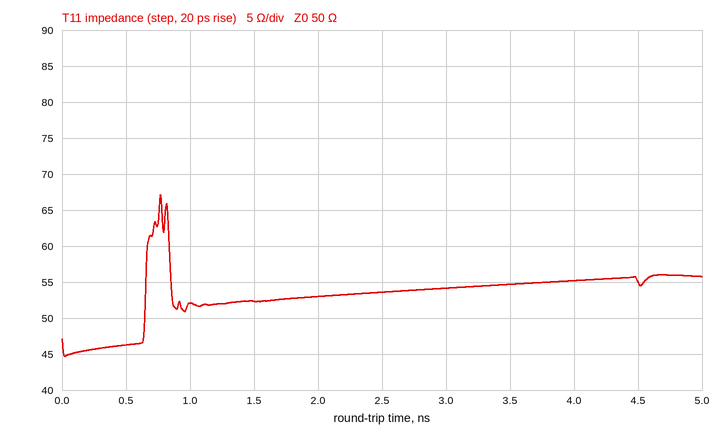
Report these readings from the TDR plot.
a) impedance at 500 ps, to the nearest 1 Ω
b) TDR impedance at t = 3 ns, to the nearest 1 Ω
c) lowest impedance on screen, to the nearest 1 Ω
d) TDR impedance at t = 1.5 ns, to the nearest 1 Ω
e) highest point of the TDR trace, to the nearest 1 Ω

46 Ω
54 Ω
45 Ω
52 Ω
67 Ω
